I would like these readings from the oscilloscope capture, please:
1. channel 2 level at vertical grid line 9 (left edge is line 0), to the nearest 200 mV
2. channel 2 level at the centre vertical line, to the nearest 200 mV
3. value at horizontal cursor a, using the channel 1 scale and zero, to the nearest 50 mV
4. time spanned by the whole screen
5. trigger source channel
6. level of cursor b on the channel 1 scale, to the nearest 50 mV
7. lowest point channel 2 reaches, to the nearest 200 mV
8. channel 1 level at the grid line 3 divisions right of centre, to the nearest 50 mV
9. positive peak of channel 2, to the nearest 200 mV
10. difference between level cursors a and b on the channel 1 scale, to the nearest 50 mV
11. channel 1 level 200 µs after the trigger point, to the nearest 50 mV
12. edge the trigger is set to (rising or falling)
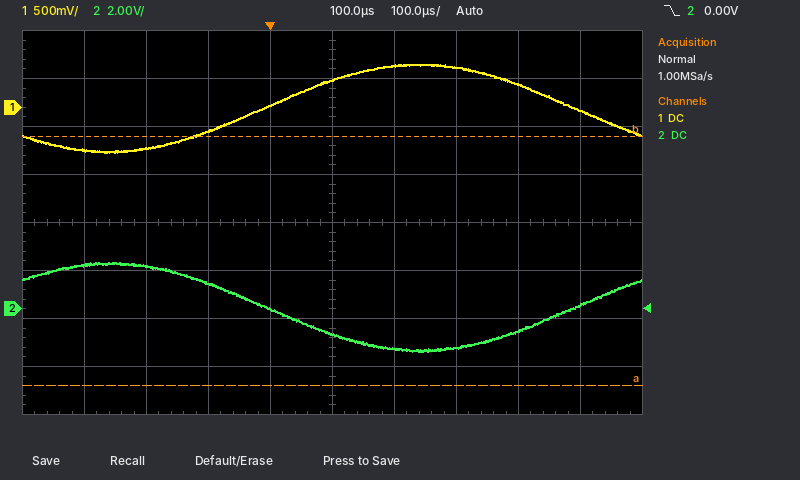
200 mV
-1.0 V
-2.90 V
1 ms
channel 2
-300 mV
-1.8 V
250 mV
2.0 V
2.60 V
450 mV
falling
